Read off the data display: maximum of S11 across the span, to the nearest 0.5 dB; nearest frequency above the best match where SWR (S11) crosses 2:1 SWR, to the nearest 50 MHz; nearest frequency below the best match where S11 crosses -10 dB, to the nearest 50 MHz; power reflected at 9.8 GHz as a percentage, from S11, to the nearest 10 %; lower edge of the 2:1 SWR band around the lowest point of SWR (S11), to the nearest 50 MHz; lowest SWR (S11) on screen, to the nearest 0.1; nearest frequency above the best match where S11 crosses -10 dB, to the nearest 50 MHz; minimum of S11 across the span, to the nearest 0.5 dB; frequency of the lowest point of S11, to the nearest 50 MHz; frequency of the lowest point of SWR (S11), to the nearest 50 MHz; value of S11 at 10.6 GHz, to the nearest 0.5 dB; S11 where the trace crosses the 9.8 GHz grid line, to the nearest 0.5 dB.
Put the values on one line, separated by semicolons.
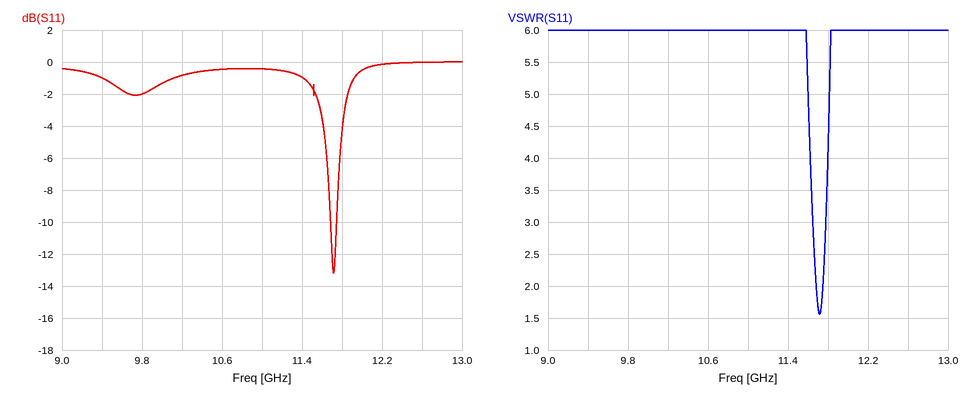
0.0 dB; 11.75 GHz; 11.70 GHz; 60 %; 11.70 GHz; 1.6; 11.75 GHz; -13.0 dB; 11.70 GHz; 11.70 GHz; -0.5 dB; -2.0 dB
